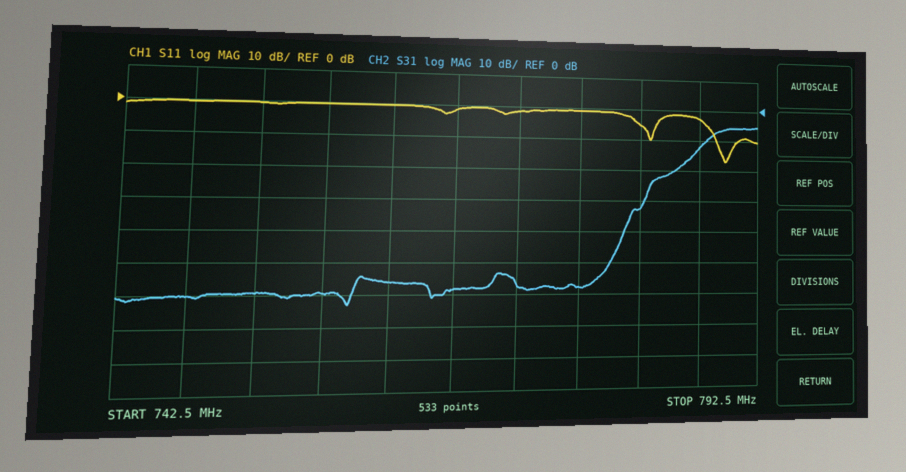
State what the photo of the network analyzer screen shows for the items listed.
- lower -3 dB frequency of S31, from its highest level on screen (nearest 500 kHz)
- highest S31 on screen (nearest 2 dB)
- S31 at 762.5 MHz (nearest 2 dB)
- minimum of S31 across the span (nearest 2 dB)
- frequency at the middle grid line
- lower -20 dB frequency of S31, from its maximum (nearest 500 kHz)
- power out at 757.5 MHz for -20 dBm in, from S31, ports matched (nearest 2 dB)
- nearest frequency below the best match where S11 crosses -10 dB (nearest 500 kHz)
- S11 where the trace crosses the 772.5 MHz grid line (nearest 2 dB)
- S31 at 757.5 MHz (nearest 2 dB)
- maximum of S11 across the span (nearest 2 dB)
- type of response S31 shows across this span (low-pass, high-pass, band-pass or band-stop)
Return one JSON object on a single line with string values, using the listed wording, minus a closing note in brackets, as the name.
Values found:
{"lower -3 dB frequency of S31, from its highest level on screen": "788.5 MHz", "highest S31 on screen": "-6 dB", "S31 at 762.5 MHz": "-56 dB", "minimum of S31 across the span": "-64 dB", "frequency at the middle grid line": "767.5 MHz", "lower -20 dB frequency of S31, from its maximum": "783.5 MHz", "power out at 757.5 MHz for -20 dBm in, from S31, ports matched": "-80 dBm", "nearest frequency below the best match where S11 crosses -10 dB": "789.0 MHz", "S11 where the trace crosses the 772.5 MHz grid line": "-2 dB", "S31 at 757.5 MHz": "-60 dB", "maximum of S11 across the span": "0 dB", "type of response S31 shows across this span": "high-pass"}
